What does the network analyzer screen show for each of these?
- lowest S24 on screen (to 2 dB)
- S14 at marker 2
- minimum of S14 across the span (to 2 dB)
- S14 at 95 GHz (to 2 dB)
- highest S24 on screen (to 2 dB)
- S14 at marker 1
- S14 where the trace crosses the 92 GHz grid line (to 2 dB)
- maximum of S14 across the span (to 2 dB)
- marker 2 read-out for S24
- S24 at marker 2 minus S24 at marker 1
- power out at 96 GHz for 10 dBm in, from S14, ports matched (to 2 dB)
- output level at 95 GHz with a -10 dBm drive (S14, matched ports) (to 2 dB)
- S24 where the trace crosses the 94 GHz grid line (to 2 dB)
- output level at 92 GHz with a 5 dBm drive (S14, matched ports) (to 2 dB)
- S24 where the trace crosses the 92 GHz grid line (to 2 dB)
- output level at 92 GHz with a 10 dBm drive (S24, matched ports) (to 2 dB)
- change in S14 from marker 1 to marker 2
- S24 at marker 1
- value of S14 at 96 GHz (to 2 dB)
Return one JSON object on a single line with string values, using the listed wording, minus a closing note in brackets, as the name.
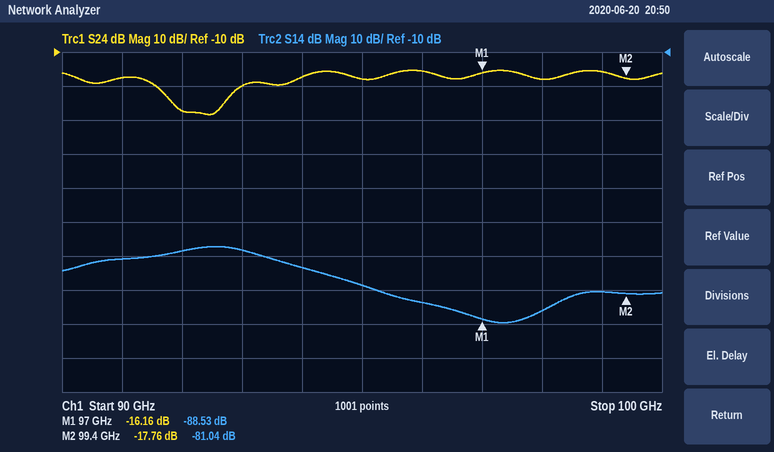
{"lowest S24 on screen": "-28 dB", "S14 at marker 2": "-81.04 dB", "minimum of S14 across the span": "-90 dB", "S14 at 95 GHz": "-78 dB", "highest S24 on screen": "-16 dB", "S14 at marker 1": "-88.53 dB", "S14 where the trace crosses the 92 GHz grid line": "-68 dB", "maximum of S14 across the span": "-68 dB", "marker 2 read-out for S24": "-17.76 dB", "S24 at marker 2 minus S24 at marker 1": "-1.60 dB", "power out at 96 GHz for 10 dBm in, from S14, ports matched": "-74 dBm", "output level at 95 GHz with a -10 dBm drive (S14, matched ports)": "-88 dBm", "S24 where the trace crosses the 94 GHz grid line": "-18 dB", "output level at 92 GHz with a 5 dBm drive (S14, matched ports)": "-64 dBm", "S24 where the trace crosses the 92 GHz grid line": "-28 dB", "output level at 92 GHz with a 10 dBm drive (S24, matched ports)": "-18 dBm", "change in S14 from marker 1 to marker 2": "7.49 dB", "S24 at marker 1": "-16.16 dB", "value of S14 at 96 GHz": "-84 dB"}
